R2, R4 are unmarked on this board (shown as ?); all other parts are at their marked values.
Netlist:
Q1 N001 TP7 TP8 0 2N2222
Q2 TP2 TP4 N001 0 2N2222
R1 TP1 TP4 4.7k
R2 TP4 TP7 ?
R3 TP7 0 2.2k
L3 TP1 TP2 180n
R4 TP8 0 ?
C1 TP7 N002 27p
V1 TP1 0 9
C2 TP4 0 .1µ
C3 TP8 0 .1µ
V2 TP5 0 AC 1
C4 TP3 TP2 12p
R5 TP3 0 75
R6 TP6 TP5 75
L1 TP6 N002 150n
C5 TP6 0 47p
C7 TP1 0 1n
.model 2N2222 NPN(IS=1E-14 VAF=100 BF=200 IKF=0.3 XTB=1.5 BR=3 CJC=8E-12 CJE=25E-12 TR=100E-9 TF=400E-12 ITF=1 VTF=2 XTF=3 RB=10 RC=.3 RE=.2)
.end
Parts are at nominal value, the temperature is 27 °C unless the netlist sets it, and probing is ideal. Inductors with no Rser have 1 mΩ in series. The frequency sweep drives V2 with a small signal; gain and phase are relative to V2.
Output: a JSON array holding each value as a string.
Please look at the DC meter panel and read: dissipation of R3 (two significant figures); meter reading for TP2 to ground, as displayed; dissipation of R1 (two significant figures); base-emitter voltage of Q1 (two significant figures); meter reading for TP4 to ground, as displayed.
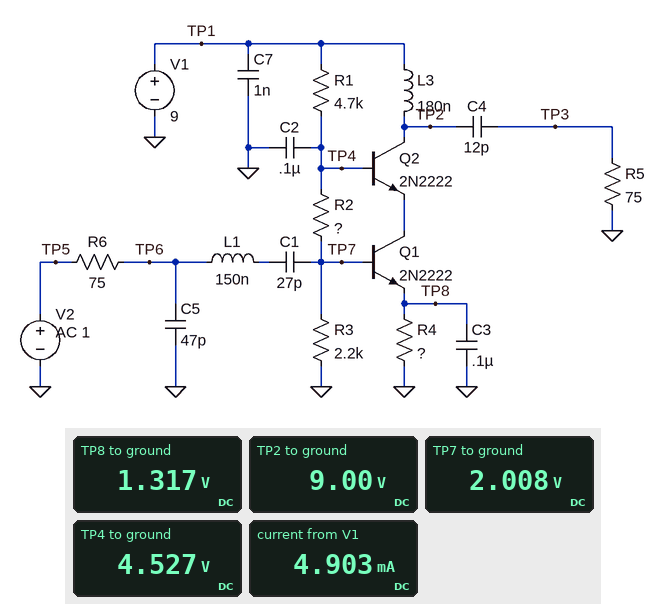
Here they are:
["1.8 mW", "9.00 V", "4.3 mW", "690 mV", "4.527 V"]
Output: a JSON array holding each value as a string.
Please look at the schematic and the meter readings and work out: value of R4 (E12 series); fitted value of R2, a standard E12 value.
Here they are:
["330 Ω", "2.7 kΩ"]
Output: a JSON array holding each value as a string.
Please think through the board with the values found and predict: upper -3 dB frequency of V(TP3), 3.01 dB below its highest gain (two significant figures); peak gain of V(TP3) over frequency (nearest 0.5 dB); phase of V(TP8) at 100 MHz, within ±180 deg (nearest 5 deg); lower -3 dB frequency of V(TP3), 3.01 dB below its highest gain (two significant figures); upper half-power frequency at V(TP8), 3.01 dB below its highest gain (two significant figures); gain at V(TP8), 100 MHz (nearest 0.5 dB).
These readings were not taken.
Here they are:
["110 MHz", "14.0 dB", "150 deg", "90 MHz", "2.0 MHz", "-64.0 dB"]
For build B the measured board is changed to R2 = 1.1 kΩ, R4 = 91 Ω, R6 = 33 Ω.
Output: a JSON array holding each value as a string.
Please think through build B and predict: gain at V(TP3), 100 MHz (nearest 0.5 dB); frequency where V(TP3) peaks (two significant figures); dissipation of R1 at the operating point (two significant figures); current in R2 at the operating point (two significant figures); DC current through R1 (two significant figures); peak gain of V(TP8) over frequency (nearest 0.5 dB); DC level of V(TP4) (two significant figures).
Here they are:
["20.5 dB", "93 MHz", "6.6 mW", "1.1 mA", "1.2 mA", "-30.0 dB", "3.4 V"]
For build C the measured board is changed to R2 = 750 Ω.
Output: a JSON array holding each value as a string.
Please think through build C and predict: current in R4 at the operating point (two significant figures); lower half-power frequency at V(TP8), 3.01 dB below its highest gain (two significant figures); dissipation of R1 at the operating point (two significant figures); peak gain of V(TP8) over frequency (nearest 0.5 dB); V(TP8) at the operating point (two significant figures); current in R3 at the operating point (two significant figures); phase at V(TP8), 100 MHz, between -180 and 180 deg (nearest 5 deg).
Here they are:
["5.5 mA", "190 kHz", "6.7 mW", "-34.5 dB", "1.8 V", "1.1 mA", "140 deg"]
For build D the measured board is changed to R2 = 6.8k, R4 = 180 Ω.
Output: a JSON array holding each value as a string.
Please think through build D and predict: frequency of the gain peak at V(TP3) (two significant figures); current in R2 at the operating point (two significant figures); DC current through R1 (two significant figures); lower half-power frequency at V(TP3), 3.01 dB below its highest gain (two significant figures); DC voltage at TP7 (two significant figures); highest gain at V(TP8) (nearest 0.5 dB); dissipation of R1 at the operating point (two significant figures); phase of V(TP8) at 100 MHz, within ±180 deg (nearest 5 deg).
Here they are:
["100 MHz", "650 µA", "670 µA", "89 MHz", "1.4 V", "-31.0 dB", "2.1 mW", "155 deg"]
